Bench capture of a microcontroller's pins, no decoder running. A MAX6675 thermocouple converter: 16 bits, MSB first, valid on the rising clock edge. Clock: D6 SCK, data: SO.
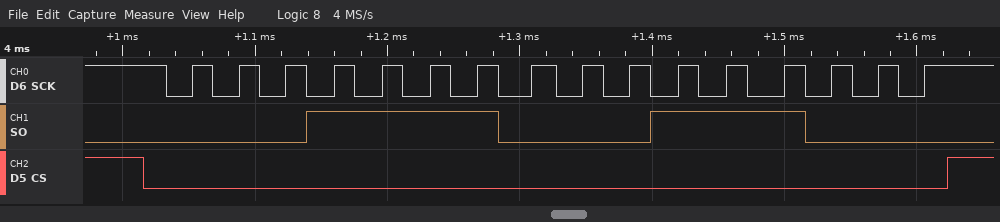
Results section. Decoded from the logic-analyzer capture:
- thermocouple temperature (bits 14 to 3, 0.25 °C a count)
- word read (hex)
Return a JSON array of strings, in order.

["241.75 °C", "0x1E38"]
